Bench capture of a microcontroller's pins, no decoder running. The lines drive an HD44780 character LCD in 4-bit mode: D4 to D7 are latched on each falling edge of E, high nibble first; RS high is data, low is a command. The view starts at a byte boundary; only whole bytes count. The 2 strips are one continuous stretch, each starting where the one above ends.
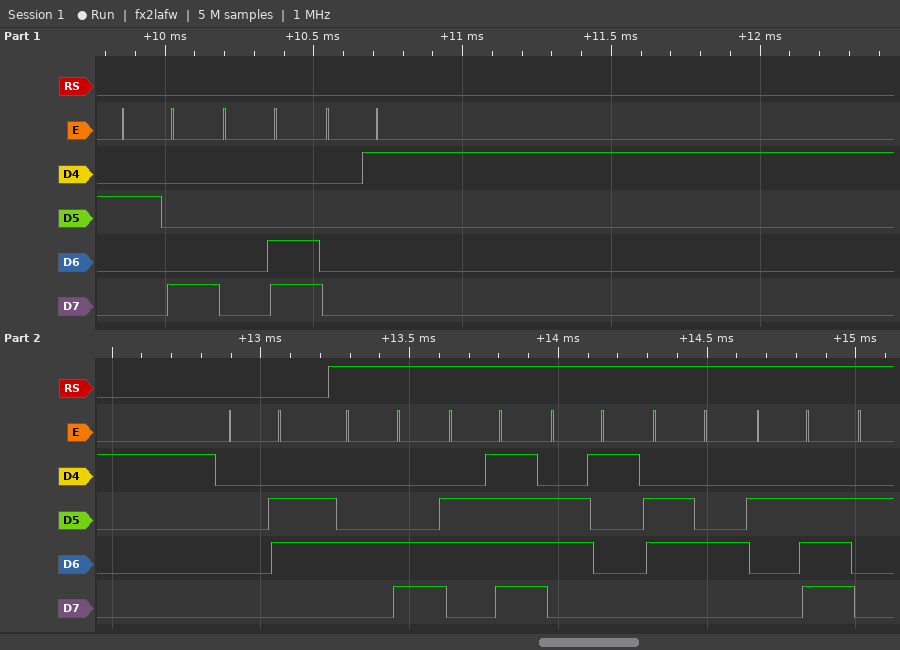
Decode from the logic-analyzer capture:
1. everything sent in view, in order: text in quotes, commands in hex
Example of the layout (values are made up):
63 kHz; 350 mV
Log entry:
0x28 0x0C 0x01 0x06 "Load."
